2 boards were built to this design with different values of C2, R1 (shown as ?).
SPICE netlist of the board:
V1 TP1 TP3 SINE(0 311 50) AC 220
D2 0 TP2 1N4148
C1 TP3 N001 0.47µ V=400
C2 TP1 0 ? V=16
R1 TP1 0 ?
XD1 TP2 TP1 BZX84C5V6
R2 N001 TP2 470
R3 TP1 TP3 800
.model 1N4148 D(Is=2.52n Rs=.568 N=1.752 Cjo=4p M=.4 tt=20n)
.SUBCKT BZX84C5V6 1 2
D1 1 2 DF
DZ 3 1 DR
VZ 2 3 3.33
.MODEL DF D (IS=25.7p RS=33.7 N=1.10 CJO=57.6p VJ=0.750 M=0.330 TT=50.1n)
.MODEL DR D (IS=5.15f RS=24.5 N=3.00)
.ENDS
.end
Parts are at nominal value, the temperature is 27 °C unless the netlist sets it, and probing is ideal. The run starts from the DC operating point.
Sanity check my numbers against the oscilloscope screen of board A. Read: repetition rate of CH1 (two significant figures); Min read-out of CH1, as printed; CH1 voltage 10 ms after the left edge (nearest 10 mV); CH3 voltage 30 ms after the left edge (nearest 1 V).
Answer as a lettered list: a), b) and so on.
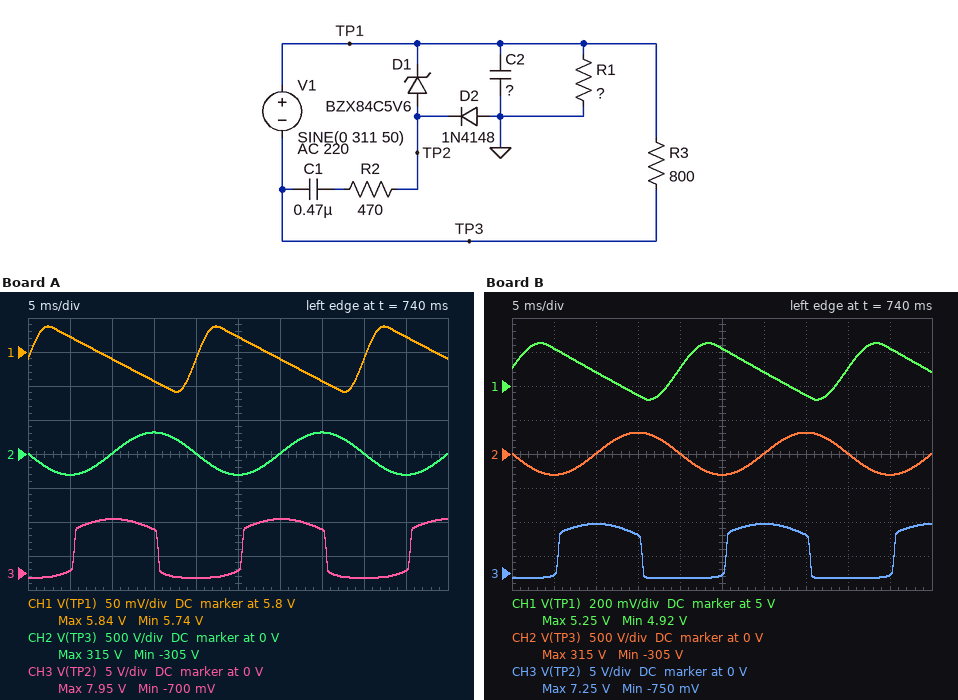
a) 50 Hz
b) 5.74 V
c) 5.79 V
d) 8 V
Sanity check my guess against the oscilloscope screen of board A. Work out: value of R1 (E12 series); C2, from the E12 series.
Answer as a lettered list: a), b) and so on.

a) 3.3 kΩ
b) 270 µF
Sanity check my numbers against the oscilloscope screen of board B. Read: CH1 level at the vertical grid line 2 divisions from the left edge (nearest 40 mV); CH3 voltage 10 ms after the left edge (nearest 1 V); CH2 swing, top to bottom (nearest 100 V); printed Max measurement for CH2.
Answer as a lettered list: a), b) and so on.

a) 5.08 V
b) 7 V
c) 600 V
d) 315 V
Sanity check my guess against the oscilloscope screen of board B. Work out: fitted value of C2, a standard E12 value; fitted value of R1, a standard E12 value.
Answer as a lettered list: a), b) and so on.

a) 330 µF
b) 560 Ω
